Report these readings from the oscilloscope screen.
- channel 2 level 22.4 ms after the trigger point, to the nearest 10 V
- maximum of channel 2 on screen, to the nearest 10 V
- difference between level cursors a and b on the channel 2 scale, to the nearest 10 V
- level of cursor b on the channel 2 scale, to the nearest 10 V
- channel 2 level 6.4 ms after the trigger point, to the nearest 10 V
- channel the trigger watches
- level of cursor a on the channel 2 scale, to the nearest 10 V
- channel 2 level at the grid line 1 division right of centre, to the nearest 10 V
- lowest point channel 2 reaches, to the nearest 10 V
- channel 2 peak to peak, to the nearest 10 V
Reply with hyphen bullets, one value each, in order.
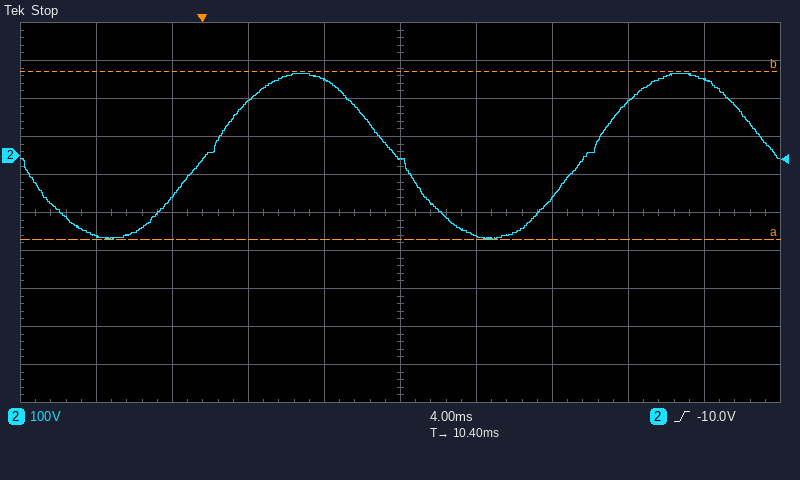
- 140 V
- 220 V
- 440 V
- 220 V
- 200 V
- channel 2
- -220 V
- -210 V
- -220 V
- 440 V
